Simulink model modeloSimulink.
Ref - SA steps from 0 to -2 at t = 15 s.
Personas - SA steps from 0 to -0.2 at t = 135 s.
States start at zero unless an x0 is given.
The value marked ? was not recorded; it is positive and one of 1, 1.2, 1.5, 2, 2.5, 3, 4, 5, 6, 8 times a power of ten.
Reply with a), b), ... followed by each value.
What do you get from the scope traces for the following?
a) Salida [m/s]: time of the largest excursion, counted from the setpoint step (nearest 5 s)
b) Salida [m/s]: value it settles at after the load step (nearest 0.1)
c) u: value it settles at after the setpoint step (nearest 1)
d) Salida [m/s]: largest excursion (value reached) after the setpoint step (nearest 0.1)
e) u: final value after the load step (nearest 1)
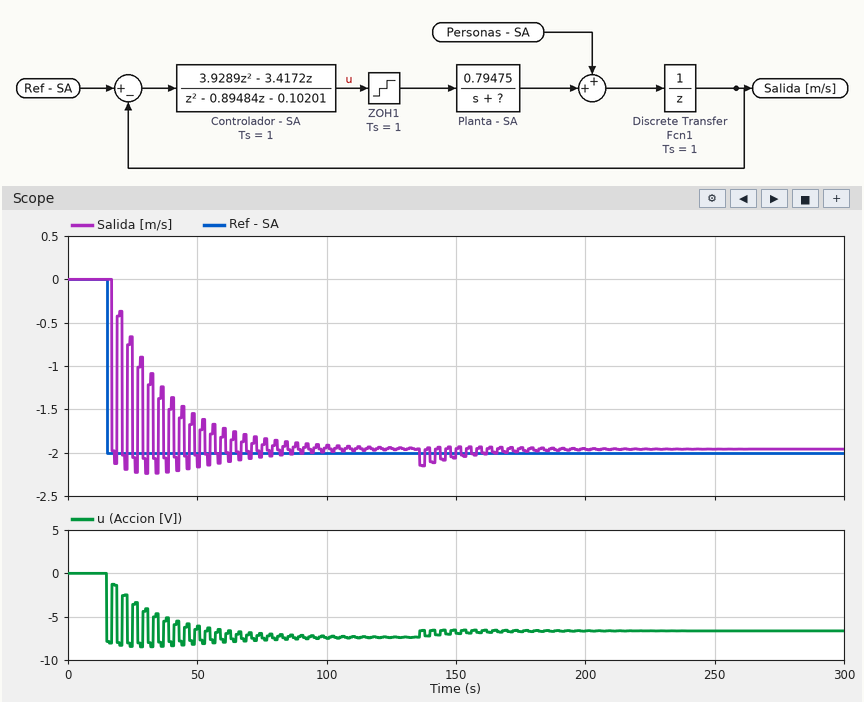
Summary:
a) 15 s
b) -2.0
c) -7
d) -2.2
e) -7
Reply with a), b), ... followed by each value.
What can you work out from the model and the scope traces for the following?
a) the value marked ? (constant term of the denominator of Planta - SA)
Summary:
a) 3
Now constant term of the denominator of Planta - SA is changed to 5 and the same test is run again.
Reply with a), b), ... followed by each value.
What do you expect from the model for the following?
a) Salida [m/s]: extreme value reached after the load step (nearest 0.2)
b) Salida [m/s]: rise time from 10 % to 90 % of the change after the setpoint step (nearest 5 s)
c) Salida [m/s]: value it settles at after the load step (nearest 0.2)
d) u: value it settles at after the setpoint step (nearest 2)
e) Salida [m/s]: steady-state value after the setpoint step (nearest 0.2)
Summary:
a) -2.2
b) 35 s
c) -2.0
d) -12
e) -2.0
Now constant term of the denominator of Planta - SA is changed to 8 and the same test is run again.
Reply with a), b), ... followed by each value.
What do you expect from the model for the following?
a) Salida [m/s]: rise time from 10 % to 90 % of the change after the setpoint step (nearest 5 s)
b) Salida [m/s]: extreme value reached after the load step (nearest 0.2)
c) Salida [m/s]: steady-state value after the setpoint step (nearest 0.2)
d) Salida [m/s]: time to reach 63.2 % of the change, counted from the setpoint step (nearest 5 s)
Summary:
a) 50 s
b) -2.0
c) -1.8
d) 20 s
